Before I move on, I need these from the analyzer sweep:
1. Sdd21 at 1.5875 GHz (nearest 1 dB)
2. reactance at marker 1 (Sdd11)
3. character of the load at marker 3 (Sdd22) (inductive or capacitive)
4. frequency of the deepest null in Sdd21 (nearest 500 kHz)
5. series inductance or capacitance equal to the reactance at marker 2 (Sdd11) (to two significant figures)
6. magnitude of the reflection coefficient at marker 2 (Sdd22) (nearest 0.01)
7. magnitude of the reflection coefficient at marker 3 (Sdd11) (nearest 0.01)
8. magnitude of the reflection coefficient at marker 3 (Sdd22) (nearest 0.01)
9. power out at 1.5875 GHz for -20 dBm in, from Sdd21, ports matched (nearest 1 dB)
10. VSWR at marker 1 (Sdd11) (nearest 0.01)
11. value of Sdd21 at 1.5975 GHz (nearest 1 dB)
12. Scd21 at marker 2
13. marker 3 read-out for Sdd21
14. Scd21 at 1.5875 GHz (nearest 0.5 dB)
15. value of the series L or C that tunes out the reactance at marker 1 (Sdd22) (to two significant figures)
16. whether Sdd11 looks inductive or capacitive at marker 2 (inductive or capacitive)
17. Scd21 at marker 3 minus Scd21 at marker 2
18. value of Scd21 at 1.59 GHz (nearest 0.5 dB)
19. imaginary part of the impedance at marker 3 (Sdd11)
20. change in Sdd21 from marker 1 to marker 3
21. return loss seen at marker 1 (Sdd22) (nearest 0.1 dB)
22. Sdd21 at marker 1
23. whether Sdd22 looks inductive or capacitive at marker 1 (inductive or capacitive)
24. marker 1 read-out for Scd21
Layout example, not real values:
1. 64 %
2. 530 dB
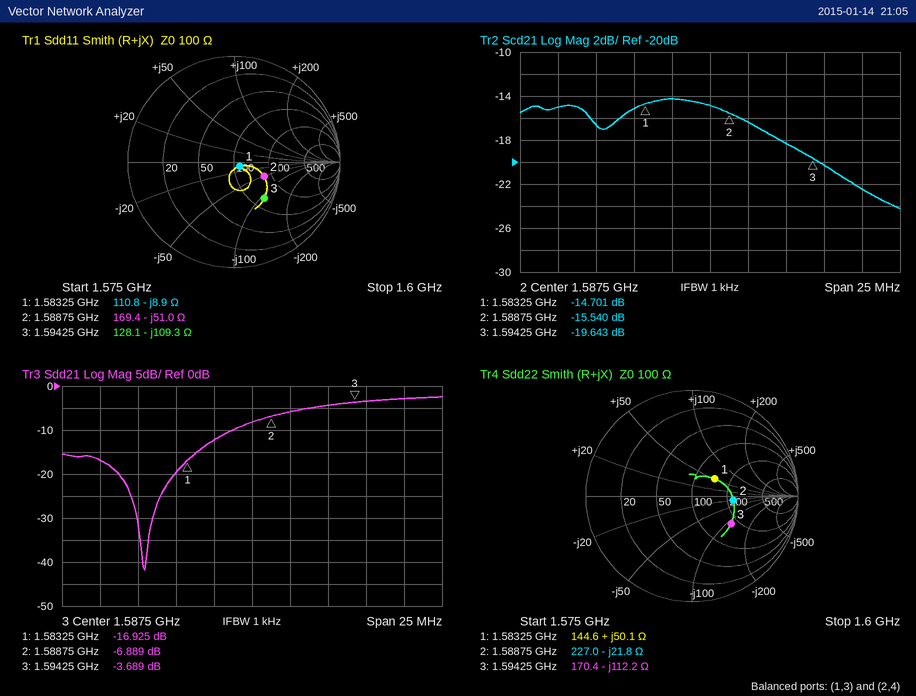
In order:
1. -8 dB
2. -8.9 Ω
3. capacitive
4. 1.5805 GHz
5. 2.0 pF
6. 0.39
7. 0.45
8. 0.45
9. -28 dBm
10. 1.14
11. -3 dB
12. -15.540 dB
13. -3.689 dB
14. -15.0 dB
15. 2.0 pF
16. capacitive
17. -4.103 dB
18. -16.5 dB
19. -109.3 Ω
20. 13.236 dB
21. 11.4 dB
22. -16.925 dB
23. inductive
24. -14.701 dB
